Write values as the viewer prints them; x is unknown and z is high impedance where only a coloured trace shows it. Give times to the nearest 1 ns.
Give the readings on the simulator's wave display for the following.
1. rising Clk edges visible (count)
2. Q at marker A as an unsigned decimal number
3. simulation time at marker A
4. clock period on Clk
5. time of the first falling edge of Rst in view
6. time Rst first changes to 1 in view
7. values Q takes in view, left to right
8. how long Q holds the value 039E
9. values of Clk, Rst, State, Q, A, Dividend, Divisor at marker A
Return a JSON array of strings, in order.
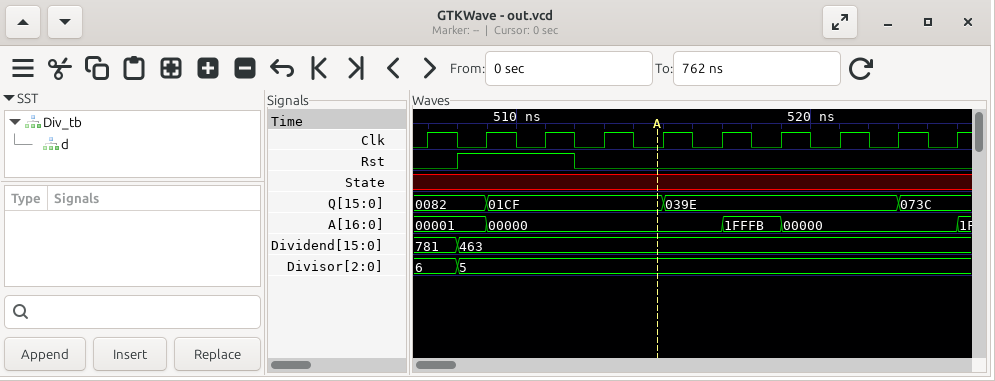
["10", "463", "515 ns", "2 ns", "512 ns", "508 ns", "0082, 01CF, 039E, 073C", "8 ns", "Clk=0, Rst=0, State=x, Q=01CF, A=00000, Dividend=463, Divisor=5"]
